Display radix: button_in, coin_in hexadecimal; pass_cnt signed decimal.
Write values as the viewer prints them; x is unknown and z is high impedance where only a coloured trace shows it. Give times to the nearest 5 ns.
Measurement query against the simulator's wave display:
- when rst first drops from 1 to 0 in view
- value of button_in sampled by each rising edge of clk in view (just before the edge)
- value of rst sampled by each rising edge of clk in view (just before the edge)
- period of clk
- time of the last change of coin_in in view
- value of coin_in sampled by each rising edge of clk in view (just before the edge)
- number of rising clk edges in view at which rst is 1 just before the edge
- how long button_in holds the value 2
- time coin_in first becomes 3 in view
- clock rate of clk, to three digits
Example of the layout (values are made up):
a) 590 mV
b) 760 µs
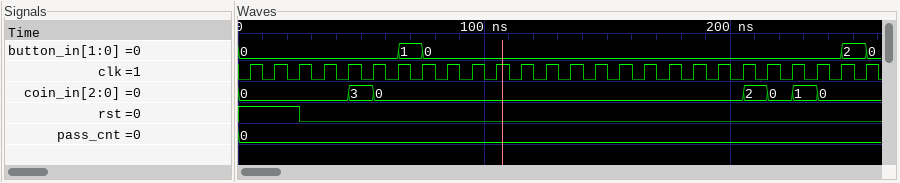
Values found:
a) 25 ns
b) 0, 0, 0, 0, 0, 0, 0, 1, 0, 0, 0, 0, 0, 0, 0, 0, 0, 0, 0, 0, 0, 0, 0, 0, 0, 2
c) 1 1 1 0 0 0 0 0 0 0 0 0 0 0 0 0 0 0 0 0 0 0 0 0 0 0
d) 10 ns
e) 235 ns
f) 0, 0, 0, 0, 0, 3, 0, 0, 0, 0, 0, 0, 0, 0, 0, 0, 0, 0, 0, 0, 0, 2, 0, 1, 0, 0
g) 3
h) 10 ns
i) 45 ns
j) 100 MHz
